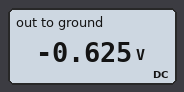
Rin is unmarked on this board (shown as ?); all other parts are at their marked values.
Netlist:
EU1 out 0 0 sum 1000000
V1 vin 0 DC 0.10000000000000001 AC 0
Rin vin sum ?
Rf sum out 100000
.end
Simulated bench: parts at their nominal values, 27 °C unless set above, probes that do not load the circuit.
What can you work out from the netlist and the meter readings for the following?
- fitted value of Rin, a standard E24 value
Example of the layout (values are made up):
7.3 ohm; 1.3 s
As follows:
16 kΩ
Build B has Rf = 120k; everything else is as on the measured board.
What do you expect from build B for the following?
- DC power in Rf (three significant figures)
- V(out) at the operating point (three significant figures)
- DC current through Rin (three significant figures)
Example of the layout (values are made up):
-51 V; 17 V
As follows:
4.69 µW; -750 mV; 6.25 µA
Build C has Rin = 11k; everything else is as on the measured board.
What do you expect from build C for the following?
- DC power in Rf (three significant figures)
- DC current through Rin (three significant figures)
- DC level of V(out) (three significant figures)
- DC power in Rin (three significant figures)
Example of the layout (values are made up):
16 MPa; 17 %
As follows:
8.26 µW; 9.09 µA; -909 mV; 909 nW
